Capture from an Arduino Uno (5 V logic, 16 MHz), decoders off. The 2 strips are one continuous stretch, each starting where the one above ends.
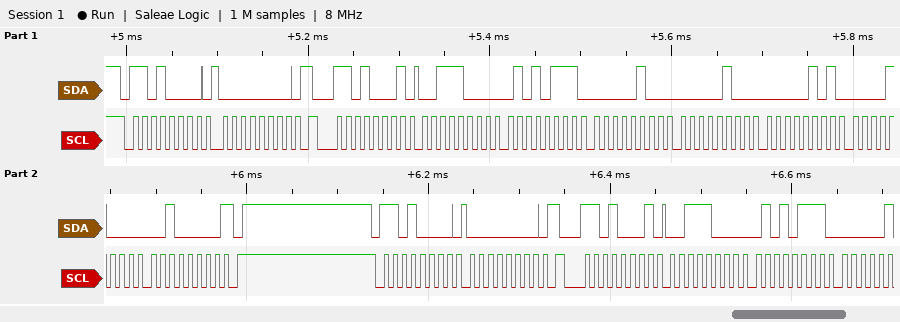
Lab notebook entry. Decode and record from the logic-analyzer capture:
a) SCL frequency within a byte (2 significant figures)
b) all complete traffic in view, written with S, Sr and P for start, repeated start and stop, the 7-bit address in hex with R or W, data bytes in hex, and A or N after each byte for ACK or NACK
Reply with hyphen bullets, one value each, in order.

- 100 kHz
- S 68W A 00 A Sr 68R A 38 A 57 A 04 A 04 A 05 A 08 A 20 N P S 68W A 00 A Sr 68R A 38 A 57 A
